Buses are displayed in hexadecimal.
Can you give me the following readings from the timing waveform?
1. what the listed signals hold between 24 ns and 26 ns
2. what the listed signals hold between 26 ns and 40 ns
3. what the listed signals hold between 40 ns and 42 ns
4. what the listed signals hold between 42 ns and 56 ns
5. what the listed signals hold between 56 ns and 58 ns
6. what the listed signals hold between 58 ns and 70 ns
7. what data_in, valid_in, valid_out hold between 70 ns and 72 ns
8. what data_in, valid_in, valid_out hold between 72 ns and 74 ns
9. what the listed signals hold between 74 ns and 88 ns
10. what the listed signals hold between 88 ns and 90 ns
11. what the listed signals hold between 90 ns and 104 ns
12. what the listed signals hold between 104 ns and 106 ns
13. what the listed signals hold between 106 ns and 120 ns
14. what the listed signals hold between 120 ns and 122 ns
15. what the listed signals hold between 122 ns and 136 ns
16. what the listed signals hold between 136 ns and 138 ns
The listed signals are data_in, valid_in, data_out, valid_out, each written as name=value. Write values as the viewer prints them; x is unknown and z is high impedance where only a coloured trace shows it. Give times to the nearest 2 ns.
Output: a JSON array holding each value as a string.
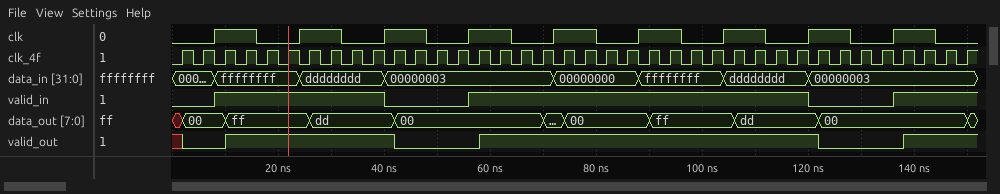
["data_in=dddddddd, valid_in=1, data_out=ff, valid_out=1", "data_in=dddddddd, valid_in=1, data_out=dd, valid_out=1", "data_in=00000003, valid_in=0, data_out=dd, valid_out=1", "data_in=00000003, valid_in=0, data_out=00, valid_out=0", "data_in=00000003, valid_in=1, data_out=00, valid_out=0", "data_in=00000003, valid_in=1, data_out=00, valid_out=1", "data_in=00000003, valid_in=1, valid_out=1", "data_in=00000000, valid_in=1, valid_out=1", "data_in=00000000, valid_in=1, data_out=00, valid_out=1", "data_in=ffffffff, valid_in=1, data_out=00, valid_out=1", "data_in=ffffffff, valid_in=1, data_out=ff, valid_out=1", "data_in=dddddddd, valid_in=1, data_out=ff, valid_out=1", "data_in=dddddddd, valid_in=1, data_out=dd, valid_out=1", "data_in=00000003, valid_in=0, data_out=dd, valid_out=1", "data_in=00000003, valid_in=0, data_out=00, valid_out=0", "data_in=00000003, valid_in=1, data_out=00, valid_out=0"]
